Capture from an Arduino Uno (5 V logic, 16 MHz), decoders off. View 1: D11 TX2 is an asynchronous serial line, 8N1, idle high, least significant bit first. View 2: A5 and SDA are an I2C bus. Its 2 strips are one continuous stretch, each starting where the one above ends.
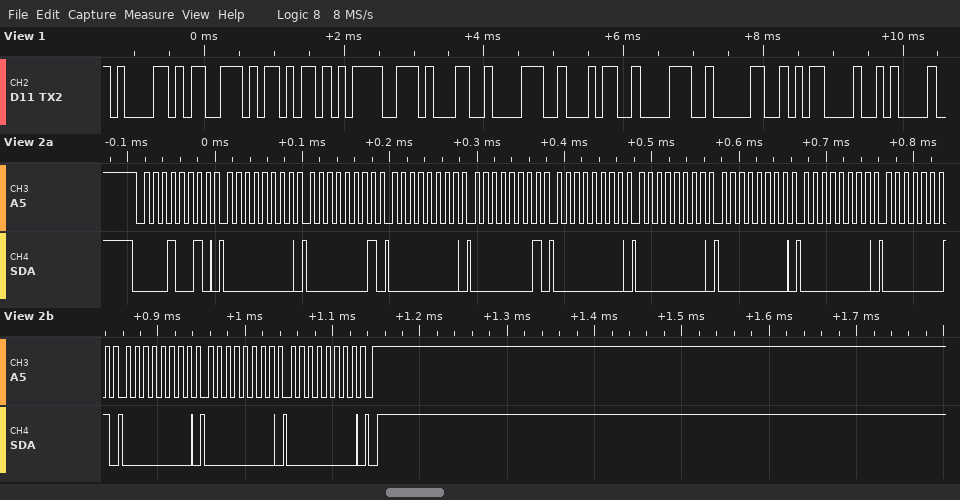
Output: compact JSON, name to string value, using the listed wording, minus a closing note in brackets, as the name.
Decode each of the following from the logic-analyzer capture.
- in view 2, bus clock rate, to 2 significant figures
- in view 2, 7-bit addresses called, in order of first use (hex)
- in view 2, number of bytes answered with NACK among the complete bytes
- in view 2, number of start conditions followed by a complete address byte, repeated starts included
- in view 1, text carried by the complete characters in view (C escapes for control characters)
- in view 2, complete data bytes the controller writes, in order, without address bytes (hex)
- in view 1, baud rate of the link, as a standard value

{"in view 2, bus clock rate, to 2 significant figures": "100 kHz", "in view 2, 7-bit addresses called, in order of first use": "0x09", "in view 2, number of bytes answered with NACK among the complete bytes": "0", "in view 2, number of start conditions followed by a complete address byte, repeated starts included": "1", "in view 1, text carried by the complete characters in view": "\"ask=18480\\r\\n\"", "in view 2, complete data bytes the controller writes, in order, without address bytes": "00 01 00 01 00 00 00 00 01 00 00 00", "in view 1, baud rate of the link, as a standard value": "9600 baud"}
